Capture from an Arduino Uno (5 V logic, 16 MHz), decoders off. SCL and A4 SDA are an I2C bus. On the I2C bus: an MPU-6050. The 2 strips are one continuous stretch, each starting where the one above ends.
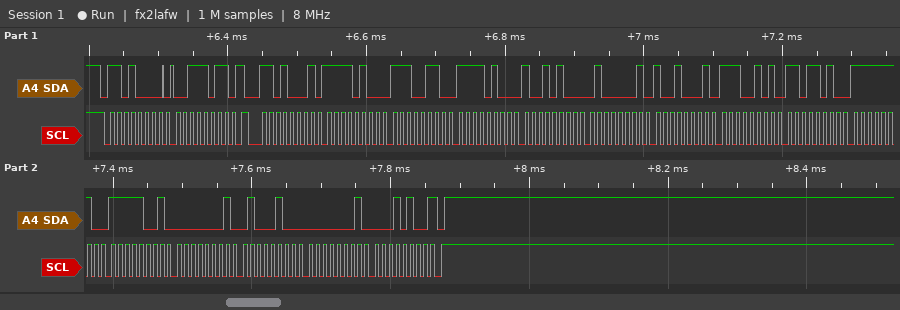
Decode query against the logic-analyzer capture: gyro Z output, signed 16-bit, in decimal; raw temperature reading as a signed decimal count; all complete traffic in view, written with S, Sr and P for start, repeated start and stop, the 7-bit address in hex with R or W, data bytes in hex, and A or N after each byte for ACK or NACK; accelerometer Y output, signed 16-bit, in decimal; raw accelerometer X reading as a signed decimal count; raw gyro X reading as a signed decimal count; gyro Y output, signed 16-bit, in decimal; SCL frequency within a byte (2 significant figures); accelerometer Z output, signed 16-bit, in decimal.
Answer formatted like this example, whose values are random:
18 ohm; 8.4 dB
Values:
276; -6694; S 68W A 3B A Sr 68R A F4 A E6 A F4 A 94 A 41 A 91 A E5 A DA A FE A F9 A 01 A 44 A 01 A 14 N P; -2924; -2842; -263; 324; 100 kHz; 16785
